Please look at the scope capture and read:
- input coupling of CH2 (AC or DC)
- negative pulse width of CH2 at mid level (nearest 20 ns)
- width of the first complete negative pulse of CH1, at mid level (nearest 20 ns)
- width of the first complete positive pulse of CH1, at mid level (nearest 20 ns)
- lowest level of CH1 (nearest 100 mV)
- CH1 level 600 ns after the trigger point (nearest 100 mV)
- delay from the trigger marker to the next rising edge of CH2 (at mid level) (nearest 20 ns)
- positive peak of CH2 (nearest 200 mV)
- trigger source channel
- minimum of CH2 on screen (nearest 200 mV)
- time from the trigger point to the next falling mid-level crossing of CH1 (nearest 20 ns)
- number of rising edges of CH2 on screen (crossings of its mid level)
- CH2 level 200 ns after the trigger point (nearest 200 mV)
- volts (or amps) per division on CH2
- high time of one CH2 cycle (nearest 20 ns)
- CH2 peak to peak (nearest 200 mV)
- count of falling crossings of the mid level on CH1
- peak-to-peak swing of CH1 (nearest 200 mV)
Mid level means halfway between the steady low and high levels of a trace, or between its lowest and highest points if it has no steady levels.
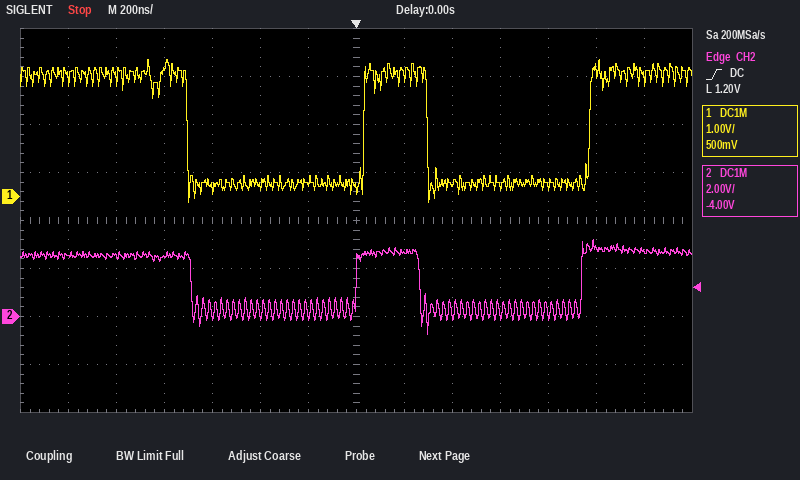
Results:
DC
680 ns
740 ns
260 ns
-100 mV
200 mV
940 ns
3.2 V
CH2
-800 mV
300 ns
2
2.6 V
2 V
260 ns
4.0 V
2
3.0 V
